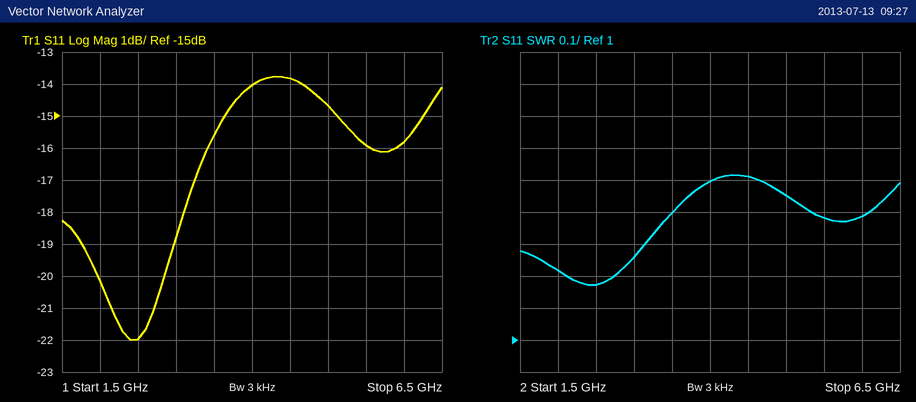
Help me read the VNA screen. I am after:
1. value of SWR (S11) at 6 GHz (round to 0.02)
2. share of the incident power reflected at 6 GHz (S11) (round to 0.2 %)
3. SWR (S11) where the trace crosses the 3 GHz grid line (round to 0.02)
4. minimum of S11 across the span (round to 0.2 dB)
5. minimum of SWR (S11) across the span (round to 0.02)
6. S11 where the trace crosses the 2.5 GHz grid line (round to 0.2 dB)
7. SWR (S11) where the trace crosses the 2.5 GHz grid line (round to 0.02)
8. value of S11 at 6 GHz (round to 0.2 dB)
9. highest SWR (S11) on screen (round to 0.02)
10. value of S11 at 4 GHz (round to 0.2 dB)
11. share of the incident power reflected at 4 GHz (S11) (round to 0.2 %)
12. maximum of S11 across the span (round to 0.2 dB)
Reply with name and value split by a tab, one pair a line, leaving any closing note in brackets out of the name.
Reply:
value of SWR (S11) at 6 GHz	1.38
share of the incident power reflected at 6 GHz (S11)	2.6 %
SWR (S11) where the trace crosses the 3 GHz grid line	1.26
minimum of S11 across the span	-22.0 dB
minimum of SWR (S11) across the span	1.18
S11 where the trace crosses the 2.5 GHz grid line	-22.0 dB
SWR (S11) where the trace crosses the 2.5 GHz grid line	1.18
value of S11 at 6 GHz	-15.8 dB
highest SWR (S11) on screen	1.52
value of S11 at 4 GHz	-14.0 dB
share of the incident power reflected at 4 GHz (S11)	4.0 %
maximum of S11 across the span	-13.8 dB
